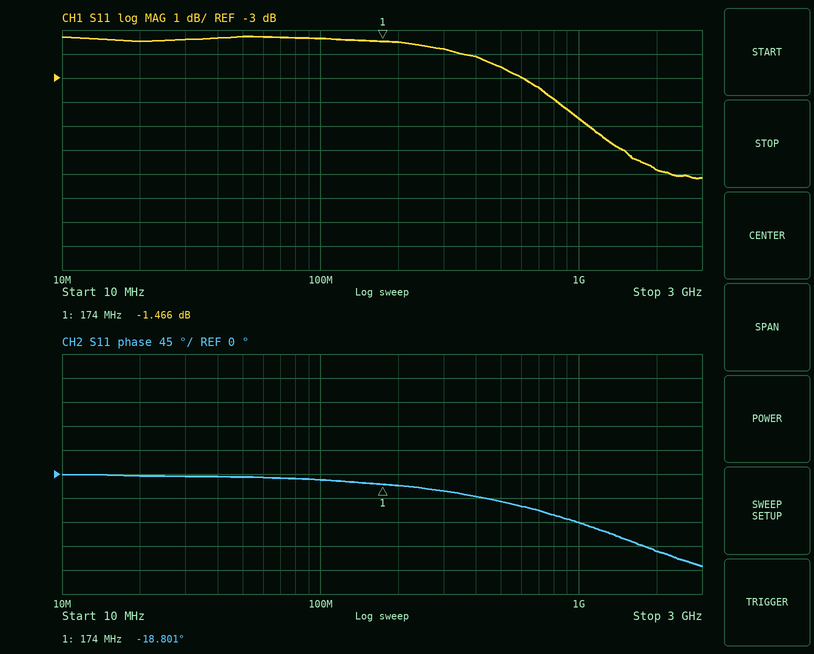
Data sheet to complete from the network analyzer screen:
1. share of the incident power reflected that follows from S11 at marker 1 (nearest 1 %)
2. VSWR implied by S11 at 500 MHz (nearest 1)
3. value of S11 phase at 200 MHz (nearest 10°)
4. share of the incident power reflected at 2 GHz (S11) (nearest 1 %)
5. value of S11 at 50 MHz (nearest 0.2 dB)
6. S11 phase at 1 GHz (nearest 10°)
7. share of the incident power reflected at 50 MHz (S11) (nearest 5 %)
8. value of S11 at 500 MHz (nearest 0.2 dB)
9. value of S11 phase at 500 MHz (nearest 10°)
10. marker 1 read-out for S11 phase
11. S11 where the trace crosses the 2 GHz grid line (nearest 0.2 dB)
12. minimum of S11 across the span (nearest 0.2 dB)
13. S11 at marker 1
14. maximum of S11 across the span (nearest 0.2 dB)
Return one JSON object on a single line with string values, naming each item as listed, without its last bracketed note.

{"share of the incident power reflected that follows from S11 at marker 1": "71 %", "VSWR implied by S11 at 500 MHz": "7", "value of S11 phase at 200 MHz": "-20°", "share of the incident power reflected at 2 GHz (S11)": "21 %", "value of S11 at 50 MHz": "-1.2 dB", "S11 phase at 1 GHz": "-90°", "share of the incident power reflected at 50 MHz (S11)": "75 %", "value of S11 at 500 MHz": "-2.6 dB", "value of S11 phase at 500 MHz": "-50°", "marker 1 read-out for S11 phase": "-18.801°", "S11 where the trace crosses the 2 GHz grid line": "-6.8 dB", "minimum of S11 across the span": "-7.2 dB", "S11 at marker 1": "-1.466 dB", "maximum of S11 across the span": "-1.2 dB"}
